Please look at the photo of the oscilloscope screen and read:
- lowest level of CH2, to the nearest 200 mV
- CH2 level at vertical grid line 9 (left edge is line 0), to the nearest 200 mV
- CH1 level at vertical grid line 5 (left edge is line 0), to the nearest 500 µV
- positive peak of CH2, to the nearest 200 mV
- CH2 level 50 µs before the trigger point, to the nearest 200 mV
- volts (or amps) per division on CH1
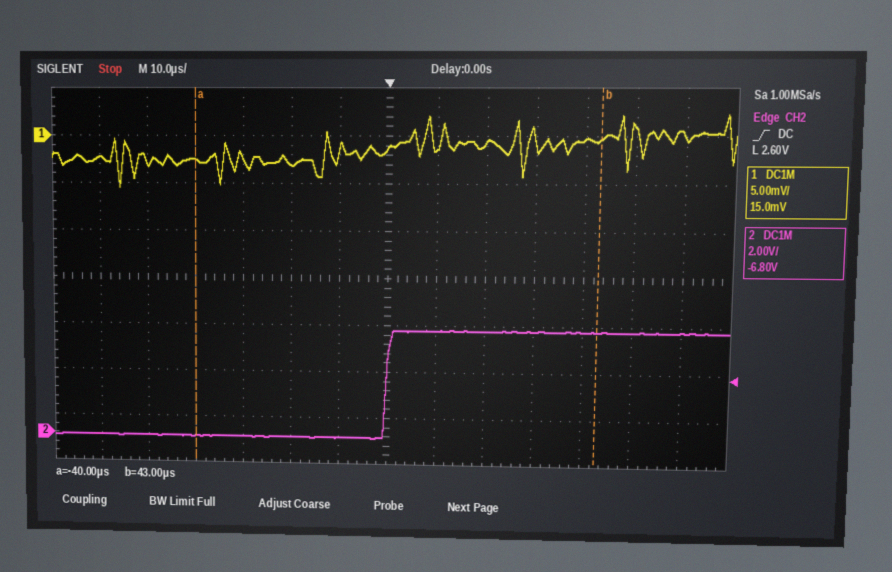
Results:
0.0 V
4.6 V
-3.0 mV
4.6 V
0.0 V
5 mV
